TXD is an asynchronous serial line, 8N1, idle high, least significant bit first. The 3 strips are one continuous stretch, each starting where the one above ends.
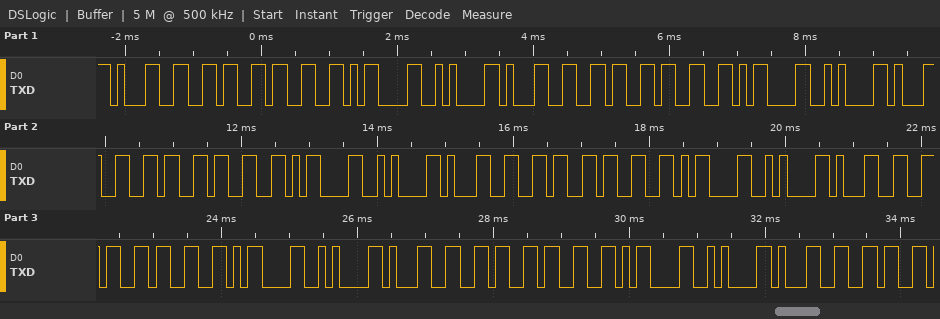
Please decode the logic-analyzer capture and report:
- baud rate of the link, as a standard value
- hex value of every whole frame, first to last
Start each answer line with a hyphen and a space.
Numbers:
- 9600 baud
- 31 36 33 0D 0A 31 36 33 0D 0A 31 36 33 0D 0A 31 36 33 0D 0A 31 36 33 0D 0A 31 36 33 0D 0A 31 36
